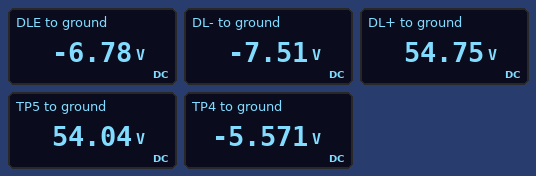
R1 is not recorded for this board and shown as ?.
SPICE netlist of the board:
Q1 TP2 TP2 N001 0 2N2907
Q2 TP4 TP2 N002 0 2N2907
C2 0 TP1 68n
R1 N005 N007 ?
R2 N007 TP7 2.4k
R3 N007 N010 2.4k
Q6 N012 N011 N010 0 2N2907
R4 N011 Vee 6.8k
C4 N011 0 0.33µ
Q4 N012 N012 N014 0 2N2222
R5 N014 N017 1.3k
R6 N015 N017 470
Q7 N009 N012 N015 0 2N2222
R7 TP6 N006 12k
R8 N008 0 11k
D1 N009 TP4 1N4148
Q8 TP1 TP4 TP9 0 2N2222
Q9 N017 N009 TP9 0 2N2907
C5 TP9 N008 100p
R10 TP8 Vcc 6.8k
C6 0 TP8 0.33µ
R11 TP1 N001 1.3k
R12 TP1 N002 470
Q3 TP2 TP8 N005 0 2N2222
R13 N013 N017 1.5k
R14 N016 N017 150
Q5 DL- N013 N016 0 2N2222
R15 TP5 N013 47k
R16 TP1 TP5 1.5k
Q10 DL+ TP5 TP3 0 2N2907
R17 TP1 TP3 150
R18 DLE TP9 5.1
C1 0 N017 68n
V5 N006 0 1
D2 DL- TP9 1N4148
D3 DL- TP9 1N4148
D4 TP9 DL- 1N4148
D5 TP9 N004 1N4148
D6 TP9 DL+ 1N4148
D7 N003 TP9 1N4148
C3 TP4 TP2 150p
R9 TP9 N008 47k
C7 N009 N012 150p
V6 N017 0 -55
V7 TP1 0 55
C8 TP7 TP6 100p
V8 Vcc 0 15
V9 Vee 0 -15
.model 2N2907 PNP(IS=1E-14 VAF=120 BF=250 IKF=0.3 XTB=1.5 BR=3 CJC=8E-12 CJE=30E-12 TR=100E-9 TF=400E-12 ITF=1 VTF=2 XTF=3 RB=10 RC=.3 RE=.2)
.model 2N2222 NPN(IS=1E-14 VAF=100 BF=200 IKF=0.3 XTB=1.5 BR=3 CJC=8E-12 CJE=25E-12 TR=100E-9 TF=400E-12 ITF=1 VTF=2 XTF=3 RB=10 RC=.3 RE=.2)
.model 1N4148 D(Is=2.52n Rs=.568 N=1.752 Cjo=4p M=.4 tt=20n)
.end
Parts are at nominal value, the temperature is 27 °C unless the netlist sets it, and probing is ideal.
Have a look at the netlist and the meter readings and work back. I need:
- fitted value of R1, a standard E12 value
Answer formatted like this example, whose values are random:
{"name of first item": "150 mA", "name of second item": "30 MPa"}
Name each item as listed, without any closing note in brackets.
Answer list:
{"fitted value of R1, a standard E12 value": "3.9 kΩ"}
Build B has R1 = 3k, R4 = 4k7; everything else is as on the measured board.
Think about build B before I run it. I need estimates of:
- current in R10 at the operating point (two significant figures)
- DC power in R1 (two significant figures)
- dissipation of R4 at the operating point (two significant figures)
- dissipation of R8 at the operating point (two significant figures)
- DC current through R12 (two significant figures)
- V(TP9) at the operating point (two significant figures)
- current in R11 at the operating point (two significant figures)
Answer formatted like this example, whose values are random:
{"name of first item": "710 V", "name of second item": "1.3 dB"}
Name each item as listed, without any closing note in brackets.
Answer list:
{"current in R10 at the operating point": "20 µA", "DC power in R1": "83 mW", "dissipation of R4 at the operating point": "1.3 µW", "dissipation of R8 at the operating point": "140 µW", "DC current through R12": "14 mA", "V(TP9) at the operating point": "-6.6 V", "current in R11 at the operating point": "5.2 mA"}
